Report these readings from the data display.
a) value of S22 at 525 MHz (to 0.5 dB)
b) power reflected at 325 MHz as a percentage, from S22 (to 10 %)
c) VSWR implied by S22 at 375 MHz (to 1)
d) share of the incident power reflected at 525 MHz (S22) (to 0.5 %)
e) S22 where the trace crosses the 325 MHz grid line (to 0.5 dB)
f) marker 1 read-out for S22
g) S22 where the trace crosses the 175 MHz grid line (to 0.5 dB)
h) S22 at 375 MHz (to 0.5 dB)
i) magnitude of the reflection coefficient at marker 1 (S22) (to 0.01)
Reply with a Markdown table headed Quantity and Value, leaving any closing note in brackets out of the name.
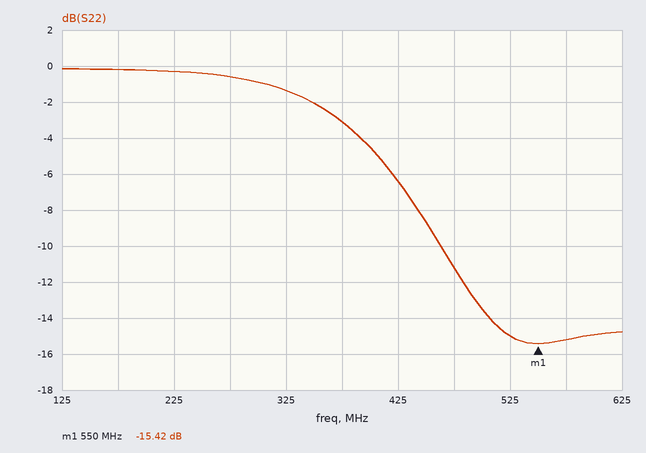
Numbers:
| Quantity | Value |
|---|---|
| value of S22 at 525 MHz | -15.0 dB |
| power reflected at 325 MHz as a percentage, from S22 | 70 % |
| VSWR implied by S22 at 375 MHz | 6 |
| share of the incident power reflected at 525 MHz (S22) | 3.0 % |
| S22 where the trace crosses the 325 MHz grid line | -1.5 dB |
| marker 1 read-out for S22 | -15.42 dB |
| S22 where the trace crosses the 175 MHz grid line | 0.0 dB |
| S22 at 375 MHz | -3.0 dB |
| magnitude of the reflection coefficient at marker 1 (S22) | 0.17 |
